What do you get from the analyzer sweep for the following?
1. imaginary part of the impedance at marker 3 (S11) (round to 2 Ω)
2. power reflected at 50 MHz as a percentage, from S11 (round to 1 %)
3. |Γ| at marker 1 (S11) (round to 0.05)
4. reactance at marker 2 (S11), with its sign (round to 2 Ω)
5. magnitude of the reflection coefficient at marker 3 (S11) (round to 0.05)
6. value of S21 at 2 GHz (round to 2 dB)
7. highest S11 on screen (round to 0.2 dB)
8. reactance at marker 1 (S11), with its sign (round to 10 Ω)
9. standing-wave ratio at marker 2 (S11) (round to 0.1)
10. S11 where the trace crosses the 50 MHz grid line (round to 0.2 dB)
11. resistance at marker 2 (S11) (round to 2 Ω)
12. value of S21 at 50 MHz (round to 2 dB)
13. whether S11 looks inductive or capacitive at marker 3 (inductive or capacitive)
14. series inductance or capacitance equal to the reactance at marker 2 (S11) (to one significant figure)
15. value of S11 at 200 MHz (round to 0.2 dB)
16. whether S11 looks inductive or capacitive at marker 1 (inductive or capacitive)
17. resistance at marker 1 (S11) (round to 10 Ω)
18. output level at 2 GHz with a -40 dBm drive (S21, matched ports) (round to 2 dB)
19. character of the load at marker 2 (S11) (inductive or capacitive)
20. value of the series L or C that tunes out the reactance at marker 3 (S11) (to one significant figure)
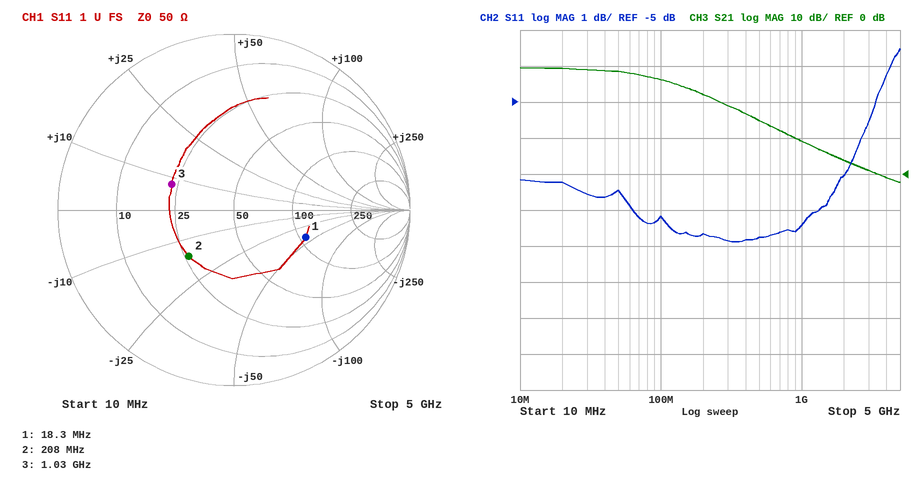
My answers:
+8 Ω
18 %
0.45
-16 Ω
0.40
4 dB
-3.6 dB
-40 Ω
2.2
-7.4 dB
26 Ω
28 dB
inductive
50 pF
-8.6 dB
capacitive
110 Ω
-36 dBm
capacitive
20 pF
